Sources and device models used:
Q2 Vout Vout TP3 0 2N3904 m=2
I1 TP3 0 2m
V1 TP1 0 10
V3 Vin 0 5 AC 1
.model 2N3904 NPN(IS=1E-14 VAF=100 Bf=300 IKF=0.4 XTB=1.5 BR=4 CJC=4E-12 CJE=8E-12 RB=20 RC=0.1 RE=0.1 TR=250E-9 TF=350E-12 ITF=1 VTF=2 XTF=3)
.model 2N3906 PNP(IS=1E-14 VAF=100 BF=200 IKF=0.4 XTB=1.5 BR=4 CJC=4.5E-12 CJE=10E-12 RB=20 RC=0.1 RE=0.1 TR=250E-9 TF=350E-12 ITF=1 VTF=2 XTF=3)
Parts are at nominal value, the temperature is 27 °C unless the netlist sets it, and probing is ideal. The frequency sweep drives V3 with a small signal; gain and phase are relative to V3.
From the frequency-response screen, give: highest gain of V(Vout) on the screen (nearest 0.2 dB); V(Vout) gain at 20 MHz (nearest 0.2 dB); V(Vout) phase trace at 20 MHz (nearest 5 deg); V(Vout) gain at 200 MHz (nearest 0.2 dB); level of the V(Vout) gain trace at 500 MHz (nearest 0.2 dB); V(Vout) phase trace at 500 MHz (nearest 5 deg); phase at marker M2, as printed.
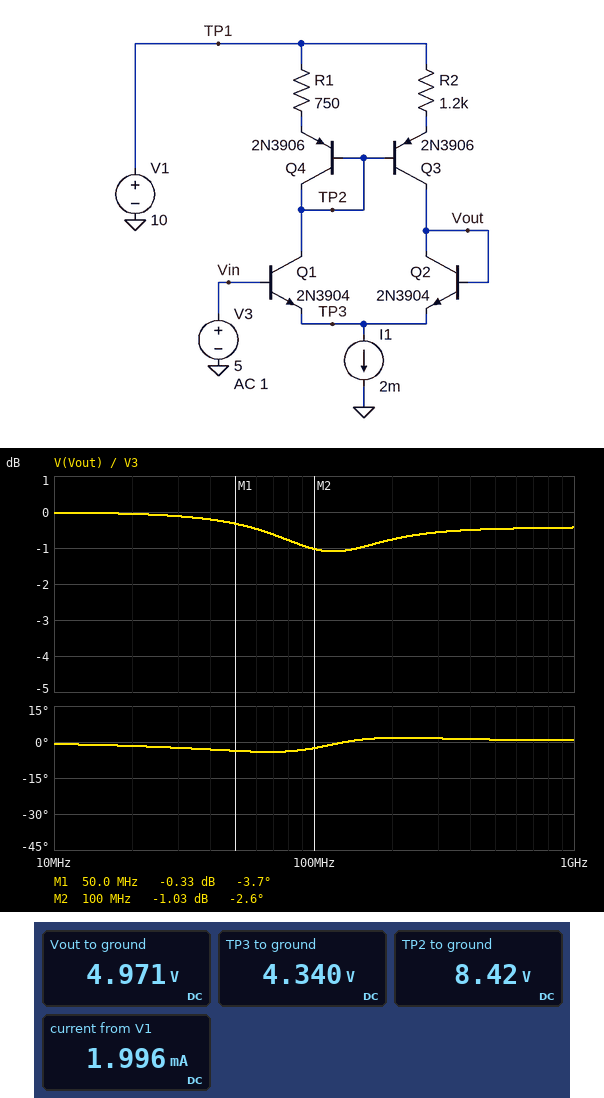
0 dB
0 dB
0 deg
-0.8 dB
-0.4 dB
0 deg
-2.6 deg
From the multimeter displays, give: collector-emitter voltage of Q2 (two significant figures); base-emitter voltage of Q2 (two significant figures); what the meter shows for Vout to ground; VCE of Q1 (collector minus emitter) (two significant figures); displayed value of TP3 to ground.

630 mV
630 mV
4.971 V
4.1 V
4.340 V
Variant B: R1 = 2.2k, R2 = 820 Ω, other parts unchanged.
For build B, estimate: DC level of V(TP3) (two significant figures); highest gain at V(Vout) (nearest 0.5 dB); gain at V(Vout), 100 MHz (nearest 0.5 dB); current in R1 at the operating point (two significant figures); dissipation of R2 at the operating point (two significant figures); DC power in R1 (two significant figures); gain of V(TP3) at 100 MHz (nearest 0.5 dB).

4.4 V
0 dB
-1.5 dB
550 µA
1.7 mW
670 µW
-1.0 dB
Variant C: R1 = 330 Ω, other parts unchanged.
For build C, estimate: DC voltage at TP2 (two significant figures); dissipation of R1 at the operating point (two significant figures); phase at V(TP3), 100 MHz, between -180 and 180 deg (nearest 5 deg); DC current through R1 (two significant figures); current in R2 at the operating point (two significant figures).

8.8 V
790 µW
-5 deg
1.5 mA
450 µA
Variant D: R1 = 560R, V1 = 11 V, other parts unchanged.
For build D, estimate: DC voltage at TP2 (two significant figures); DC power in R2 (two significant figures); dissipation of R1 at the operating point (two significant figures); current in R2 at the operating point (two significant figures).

9.6 V
500 µW
1.0 mW
650 µA
